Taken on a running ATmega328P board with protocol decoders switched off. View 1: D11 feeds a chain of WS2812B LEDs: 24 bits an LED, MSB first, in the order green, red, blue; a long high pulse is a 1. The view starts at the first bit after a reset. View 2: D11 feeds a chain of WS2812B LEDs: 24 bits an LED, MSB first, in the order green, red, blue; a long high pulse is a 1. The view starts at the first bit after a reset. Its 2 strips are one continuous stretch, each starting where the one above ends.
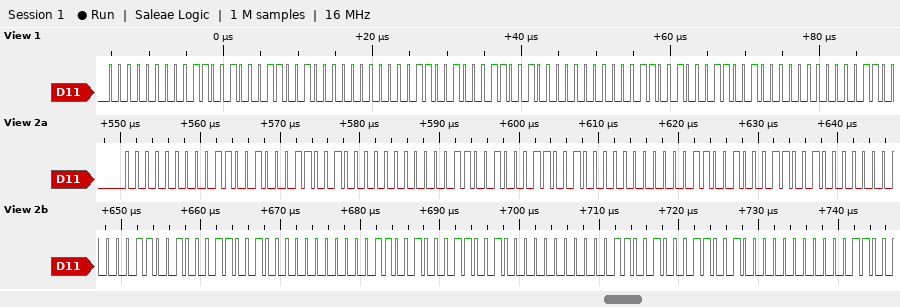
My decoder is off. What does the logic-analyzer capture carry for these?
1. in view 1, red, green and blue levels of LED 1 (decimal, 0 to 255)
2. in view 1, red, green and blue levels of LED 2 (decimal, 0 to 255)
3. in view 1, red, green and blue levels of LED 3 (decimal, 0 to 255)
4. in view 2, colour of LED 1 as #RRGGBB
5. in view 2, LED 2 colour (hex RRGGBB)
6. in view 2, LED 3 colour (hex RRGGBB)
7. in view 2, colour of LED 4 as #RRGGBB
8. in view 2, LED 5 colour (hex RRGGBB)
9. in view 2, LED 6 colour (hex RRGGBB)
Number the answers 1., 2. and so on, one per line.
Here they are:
1. 100, 0, 100
2. 100, 0, 100
3. 100, 0, 100
4. #640064
5. #640064
6. #640064
7. #640064
8. #640064
9. #640064
